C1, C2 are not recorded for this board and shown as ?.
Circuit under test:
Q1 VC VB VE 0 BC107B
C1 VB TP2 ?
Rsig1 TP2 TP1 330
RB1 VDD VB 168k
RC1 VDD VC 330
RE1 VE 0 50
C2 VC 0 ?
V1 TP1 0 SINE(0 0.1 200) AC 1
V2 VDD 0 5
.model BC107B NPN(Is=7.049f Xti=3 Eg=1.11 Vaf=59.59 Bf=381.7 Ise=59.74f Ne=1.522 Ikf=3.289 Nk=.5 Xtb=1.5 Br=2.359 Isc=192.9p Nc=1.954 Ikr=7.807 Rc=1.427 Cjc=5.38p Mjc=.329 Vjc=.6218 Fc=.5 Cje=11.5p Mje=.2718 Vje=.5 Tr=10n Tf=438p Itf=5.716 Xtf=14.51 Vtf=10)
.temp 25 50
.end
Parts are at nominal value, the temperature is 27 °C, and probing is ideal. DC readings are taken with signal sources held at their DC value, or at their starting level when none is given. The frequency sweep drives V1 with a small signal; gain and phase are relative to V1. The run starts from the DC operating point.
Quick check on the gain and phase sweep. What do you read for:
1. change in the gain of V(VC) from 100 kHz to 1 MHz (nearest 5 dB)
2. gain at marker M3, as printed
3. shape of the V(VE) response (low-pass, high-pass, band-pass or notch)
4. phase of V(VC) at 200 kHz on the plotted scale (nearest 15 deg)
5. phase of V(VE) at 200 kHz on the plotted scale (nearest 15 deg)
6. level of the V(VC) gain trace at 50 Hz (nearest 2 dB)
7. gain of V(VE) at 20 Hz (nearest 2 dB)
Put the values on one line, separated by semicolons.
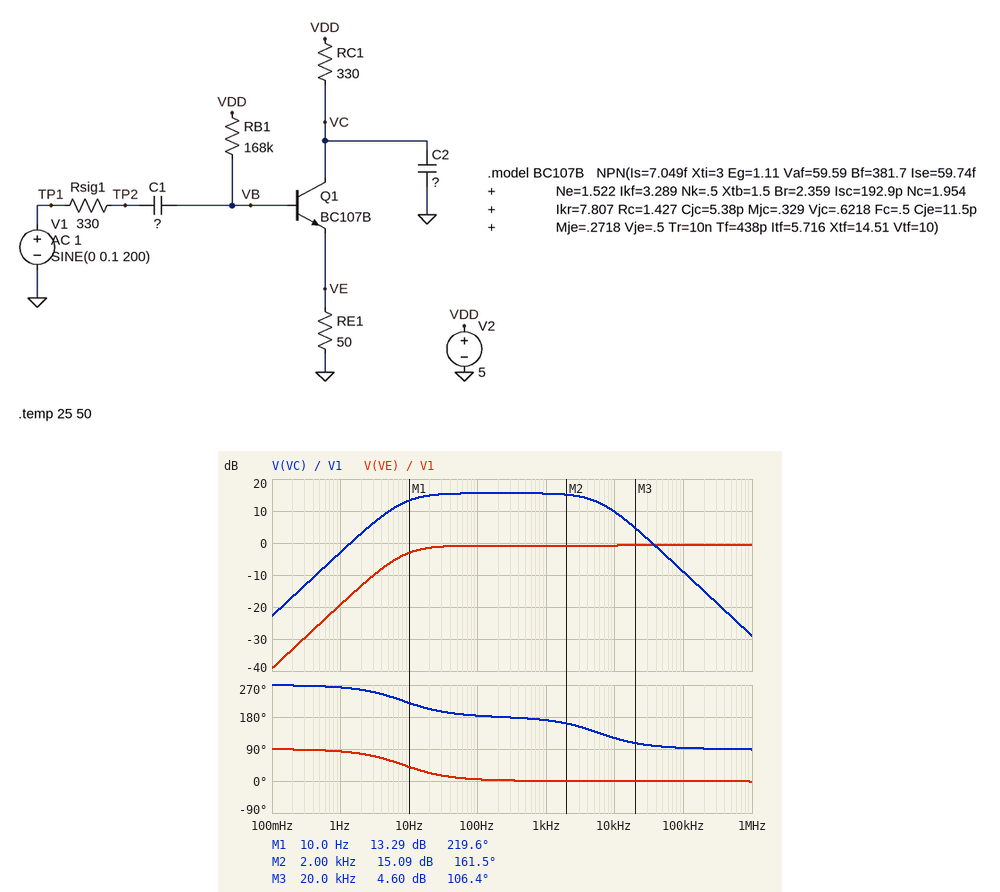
-20 dB; 4.60 dB; high-pass; 90 deg; 0 deg; 16 dB; -2 dB
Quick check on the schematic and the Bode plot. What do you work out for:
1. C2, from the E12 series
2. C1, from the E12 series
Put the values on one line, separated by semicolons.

82 nF; 1.2 µF
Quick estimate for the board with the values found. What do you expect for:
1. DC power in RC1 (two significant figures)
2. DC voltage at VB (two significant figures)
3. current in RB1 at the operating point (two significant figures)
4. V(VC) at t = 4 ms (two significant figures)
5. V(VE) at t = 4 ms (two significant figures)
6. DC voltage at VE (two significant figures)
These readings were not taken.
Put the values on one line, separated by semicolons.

18 mW; 1.1 V; 23 µA; 3.2 V; 280 mV; 370 mV
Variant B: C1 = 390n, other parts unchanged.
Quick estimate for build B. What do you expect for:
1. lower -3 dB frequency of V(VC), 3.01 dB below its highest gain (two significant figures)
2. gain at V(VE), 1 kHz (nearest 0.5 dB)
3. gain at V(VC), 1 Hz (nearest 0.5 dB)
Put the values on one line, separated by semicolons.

25 Hz; -1.0 dB; -12.5 dB
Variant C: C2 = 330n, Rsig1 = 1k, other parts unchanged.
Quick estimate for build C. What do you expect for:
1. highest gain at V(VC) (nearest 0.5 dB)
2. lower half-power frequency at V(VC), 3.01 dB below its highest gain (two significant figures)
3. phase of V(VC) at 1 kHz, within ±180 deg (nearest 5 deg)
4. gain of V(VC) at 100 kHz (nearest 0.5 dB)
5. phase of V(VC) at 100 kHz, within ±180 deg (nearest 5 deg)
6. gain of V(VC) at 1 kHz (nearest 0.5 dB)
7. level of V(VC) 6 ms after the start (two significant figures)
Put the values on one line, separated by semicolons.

15.0 dB; 7.9 Hz; 145 deg; -21.5 dB; 90 deg; 13.5 dB; 2.1 V
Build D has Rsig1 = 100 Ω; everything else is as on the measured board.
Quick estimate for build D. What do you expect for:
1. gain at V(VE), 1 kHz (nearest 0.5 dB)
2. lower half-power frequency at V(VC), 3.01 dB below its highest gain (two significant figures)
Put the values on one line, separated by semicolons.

-0.5 dB; 8.4 Hz
